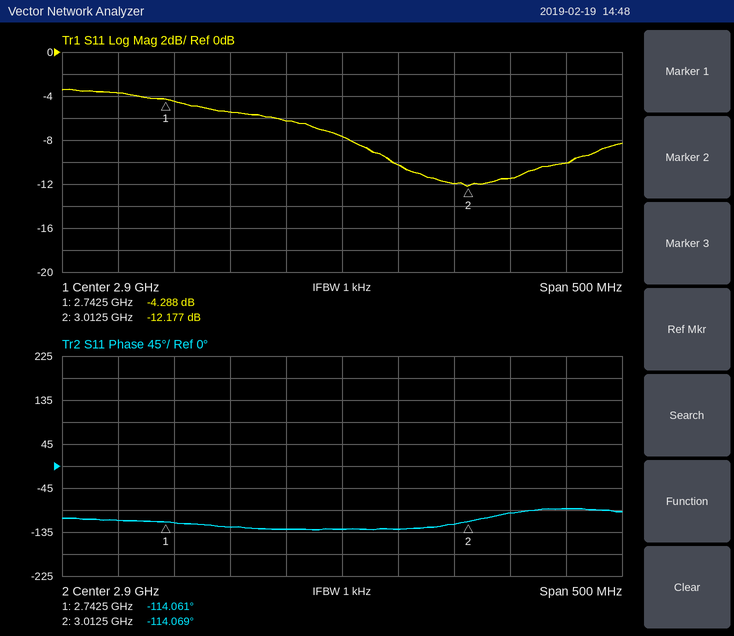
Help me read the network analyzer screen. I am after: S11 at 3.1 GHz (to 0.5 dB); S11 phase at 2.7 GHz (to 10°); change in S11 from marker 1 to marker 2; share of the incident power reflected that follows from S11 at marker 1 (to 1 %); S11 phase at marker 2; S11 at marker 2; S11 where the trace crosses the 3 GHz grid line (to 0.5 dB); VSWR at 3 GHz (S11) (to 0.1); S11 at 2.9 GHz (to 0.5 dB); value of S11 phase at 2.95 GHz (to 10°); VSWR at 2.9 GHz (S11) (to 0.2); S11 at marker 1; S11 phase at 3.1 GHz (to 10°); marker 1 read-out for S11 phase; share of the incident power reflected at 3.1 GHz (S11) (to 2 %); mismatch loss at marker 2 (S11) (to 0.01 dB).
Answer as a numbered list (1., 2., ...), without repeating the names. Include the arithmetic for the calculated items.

1. -10.0 dB
2. -110°
3. -12.177 − (-4.288) = -7.889 dB
4. 10^(-4.288/10) ≈ 37 %
5. -114.069°
6. -12.177 dB
7. -12.0 dB
8. |Γ| = 10^(-12/20) = 0.2512; VSWR = (1 + 0.2512)/(1 − 0.2512) ≈ 1.7
9. -7.5 dB
10. -130°
11. |Γ| = 10^(-7.5/20) = 0.4217; VSWR = (1 + 0.4217)/(1 − 0.4217) ≈ 2.46, so 2.4 to the nearest 0.2
12. -4.288 dB
13. -90°
14. -114.061°
15. 10^(-10/10) ≈ 10 %
16. −10 log10(1 − 10^(-12.177/10)) ≈ 0.27 dB
